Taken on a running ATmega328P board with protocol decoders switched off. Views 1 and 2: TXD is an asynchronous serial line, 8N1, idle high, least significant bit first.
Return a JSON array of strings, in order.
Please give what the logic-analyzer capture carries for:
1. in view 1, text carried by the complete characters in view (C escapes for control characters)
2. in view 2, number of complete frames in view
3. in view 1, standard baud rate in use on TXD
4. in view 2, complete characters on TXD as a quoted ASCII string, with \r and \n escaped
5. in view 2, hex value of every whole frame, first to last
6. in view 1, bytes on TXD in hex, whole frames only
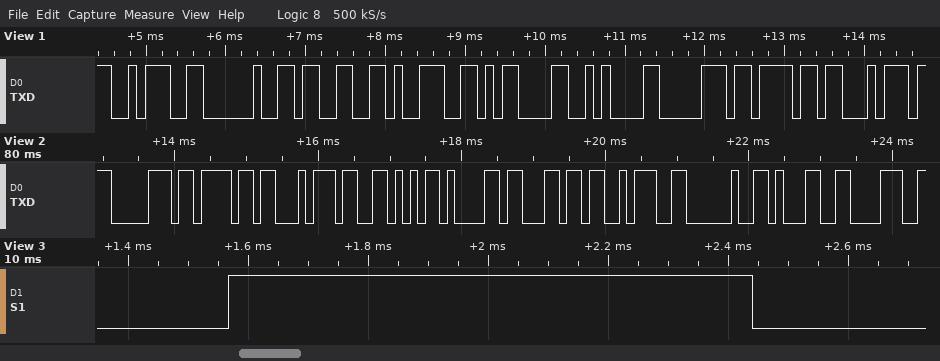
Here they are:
["\": 39\\r\\npot\"", "10", "9600 baud", "\"potVal: 18\"", "70 6F 74 56 61 6C 3A 20 31 38", "3A 20 33 39 0D 0A 70 6F 74"]
